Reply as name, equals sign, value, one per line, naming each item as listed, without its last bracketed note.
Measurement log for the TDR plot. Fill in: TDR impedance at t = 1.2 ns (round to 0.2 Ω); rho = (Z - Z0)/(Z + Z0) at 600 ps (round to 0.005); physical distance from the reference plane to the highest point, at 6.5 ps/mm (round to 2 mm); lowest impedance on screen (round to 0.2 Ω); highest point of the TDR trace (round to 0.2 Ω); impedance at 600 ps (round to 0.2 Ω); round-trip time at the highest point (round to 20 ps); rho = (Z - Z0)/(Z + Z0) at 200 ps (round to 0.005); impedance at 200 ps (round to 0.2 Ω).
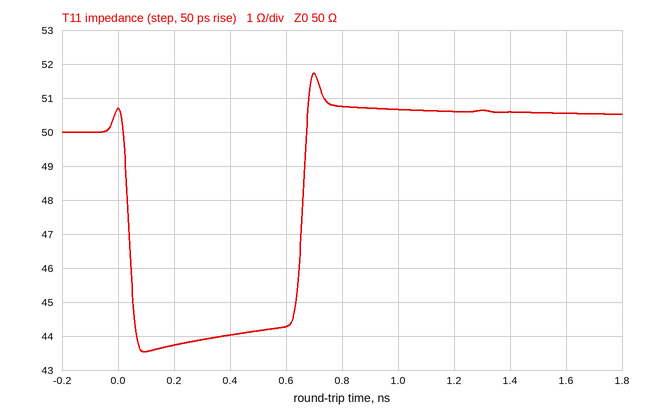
TDR impedance at t = 1.2 ns = 50.6 Ω
rho = (Z - Z0)/(Z + Z0) at 600 ps = -0.060
physical distance from the reference plane to the highest point, at 6.5 ps/mm = 54 mm
lowest impedance on screen = 43.6 Ω
highest point of the TDR trace = 51.8 Ω
impedance at 600 ps = 44.2 Ω
round-trip time at the highest point = 700 ps
rho = (Z - Z0)/(Z + Z0) at 200 ps = -0.065
impedance at 200 ps = 43.8 Ω
